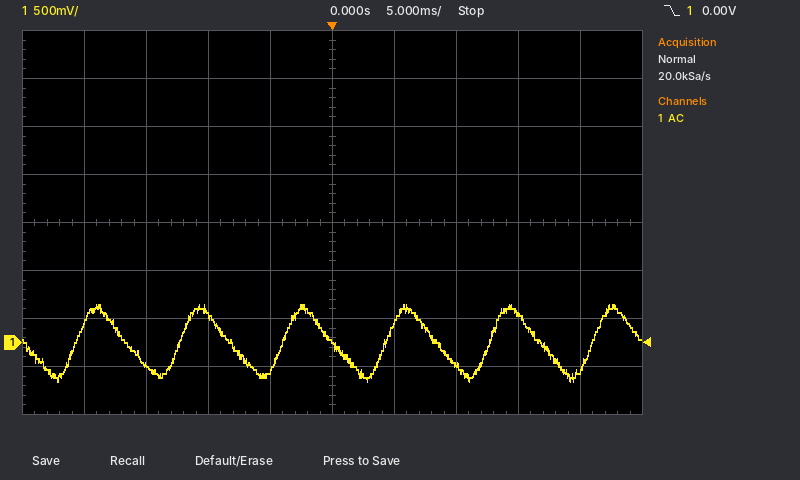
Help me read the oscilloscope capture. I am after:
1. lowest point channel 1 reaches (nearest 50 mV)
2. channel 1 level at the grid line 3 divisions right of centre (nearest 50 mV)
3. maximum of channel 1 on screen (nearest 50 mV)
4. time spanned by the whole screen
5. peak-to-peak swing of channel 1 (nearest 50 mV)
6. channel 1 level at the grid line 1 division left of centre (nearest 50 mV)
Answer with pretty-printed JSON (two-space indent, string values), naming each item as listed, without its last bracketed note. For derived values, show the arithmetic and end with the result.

{
  "lowest point channel 1 reaches": "-400 mV",
  "channel 1 level at the grid line 3 divisions right of centre": "300 mV",
  "maximum of channel 1 on screen": "400 mV",
  "time spanned by the whole screen": "50 ms",
  "peak-to-peak swing of channel 1": "400 mV − (-400 mV) = 800 mV",
  "channel 1 level at the grid line 1 division left of centre": "-300 mV"
}
